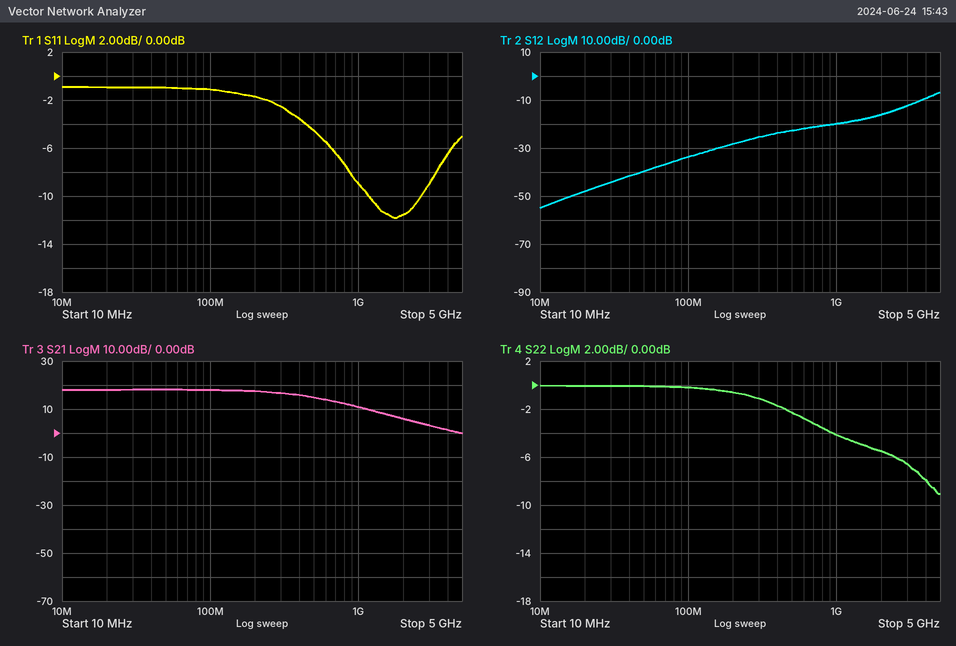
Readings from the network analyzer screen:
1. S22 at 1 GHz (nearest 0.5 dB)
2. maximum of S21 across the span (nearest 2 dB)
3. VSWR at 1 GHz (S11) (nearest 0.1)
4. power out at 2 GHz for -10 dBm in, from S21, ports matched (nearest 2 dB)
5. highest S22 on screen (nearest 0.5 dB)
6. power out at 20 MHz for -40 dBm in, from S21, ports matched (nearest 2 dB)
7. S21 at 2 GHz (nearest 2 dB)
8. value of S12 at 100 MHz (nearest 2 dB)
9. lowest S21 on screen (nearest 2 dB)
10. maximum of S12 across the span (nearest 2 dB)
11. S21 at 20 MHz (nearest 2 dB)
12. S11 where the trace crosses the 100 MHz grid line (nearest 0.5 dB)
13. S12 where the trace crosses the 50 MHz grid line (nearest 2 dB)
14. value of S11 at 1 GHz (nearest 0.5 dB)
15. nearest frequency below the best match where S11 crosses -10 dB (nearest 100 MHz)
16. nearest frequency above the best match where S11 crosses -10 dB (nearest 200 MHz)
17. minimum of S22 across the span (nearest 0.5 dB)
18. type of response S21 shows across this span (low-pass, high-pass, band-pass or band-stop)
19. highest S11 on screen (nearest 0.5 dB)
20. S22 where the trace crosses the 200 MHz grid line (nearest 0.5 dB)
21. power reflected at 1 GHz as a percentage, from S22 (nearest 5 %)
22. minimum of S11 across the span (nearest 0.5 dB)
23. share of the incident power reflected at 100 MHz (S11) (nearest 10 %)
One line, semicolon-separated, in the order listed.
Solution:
-4.0 dB; 18 dB; 2.1; -4 dBm; 0.0 dB; -22 dBm; 6 dB; -34 dB; 0 dB; -6 dB; 18 dB; -1.0 dB; -40 dB; -9.0 dB; 1.2 GHz; 2.6 GHz; -9.0 dB; low-pass; -1.0 dB; -0.5 dB; 40 %; -12.0 dB; 80 %
